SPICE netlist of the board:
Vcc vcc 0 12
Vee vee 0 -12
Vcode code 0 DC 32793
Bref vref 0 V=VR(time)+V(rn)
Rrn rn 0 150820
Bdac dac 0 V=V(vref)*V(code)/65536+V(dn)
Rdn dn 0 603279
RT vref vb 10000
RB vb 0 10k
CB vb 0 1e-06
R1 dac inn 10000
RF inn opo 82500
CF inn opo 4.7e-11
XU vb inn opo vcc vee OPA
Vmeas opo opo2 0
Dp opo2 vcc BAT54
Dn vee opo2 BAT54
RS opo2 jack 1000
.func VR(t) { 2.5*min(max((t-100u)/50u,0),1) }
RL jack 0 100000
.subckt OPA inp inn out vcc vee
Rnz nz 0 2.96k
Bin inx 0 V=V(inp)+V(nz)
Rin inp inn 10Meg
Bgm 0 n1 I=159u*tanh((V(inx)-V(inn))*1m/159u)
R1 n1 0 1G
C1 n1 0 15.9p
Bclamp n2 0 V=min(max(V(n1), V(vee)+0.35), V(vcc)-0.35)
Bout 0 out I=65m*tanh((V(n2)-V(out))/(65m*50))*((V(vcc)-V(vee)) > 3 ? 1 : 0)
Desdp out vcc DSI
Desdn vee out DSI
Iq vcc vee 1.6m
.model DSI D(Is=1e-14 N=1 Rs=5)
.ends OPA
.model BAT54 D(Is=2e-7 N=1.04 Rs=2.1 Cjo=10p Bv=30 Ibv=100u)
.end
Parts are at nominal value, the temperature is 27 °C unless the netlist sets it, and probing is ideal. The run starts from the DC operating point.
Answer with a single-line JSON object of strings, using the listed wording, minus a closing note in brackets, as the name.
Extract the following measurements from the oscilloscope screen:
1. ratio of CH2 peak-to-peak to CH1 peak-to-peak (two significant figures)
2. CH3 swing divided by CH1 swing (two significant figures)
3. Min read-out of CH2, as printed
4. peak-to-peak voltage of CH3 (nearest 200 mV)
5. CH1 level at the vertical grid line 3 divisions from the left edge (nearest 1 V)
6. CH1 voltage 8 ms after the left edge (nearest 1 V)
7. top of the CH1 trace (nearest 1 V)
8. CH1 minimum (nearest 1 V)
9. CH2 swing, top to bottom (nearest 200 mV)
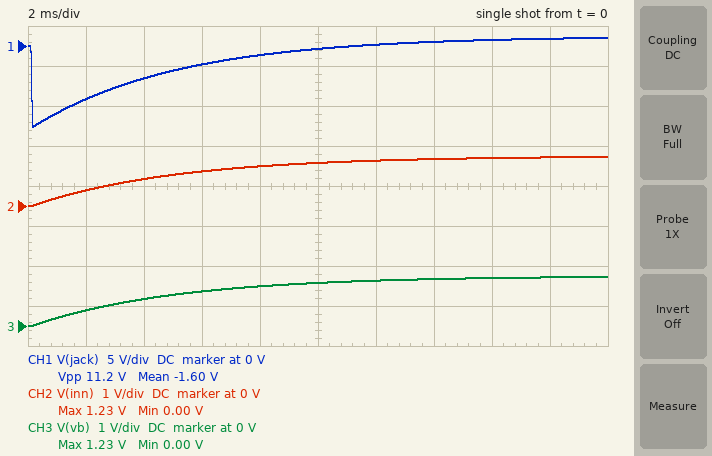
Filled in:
{"ratio of CH2 peak-to-peak to CH1 peak-to-peak": "0.11", "CH3 swing divided by CH1 swing": "0.11", "Min read-out of CH2, as printed": "0.00 V", "peak-to-peak voltage of CH3": "1.2 V", "CH1 level at the vertical grid line 3 divisions from the left edge": "-2 V", "CH1 voltage 8 ms after the left edge": "-1 V", "top of the CH1 trace": "1 V", "CH1 minimum": "-10 V", "CH2 swing, top to bottom": "1.2 V"}
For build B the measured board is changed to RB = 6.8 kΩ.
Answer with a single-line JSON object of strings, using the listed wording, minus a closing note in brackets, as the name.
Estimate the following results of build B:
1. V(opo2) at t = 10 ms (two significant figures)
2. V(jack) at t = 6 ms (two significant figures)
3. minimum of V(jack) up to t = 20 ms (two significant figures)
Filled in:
{"V(opo2) at t = 10 ms": "-1.8 V", "V(jack) at t = 6 ms": "-3.1 V", "minimum of V(jack) up to t = 20 ms": "-10 V"}
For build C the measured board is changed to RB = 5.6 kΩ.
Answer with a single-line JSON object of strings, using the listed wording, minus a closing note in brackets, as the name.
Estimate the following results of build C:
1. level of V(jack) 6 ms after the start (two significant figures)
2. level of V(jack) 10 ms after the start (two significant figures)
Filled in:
{"level of V(jack) 6 ms after the start": "-3.6 V", "level of V(jack) 10 ms after the start": "-2.5 V"}
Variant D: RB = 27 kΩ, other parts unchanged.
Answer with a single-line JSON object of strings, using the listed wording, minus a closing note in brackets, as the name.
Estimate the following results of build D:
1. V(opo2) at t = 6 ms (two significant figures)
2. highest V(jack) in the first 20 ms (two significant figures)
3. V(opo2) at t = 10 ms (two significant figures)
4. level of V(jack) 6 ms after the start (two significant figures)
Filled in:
{"V(opo2) at t = 6 ms": "-990 mV", "highest V(jack) in the first 20 ms": "5.4 V", "V(opo2) at t = 10 ms": "2.2 V", "level of V(jack) 6 ms after the start": "-980 mV"}
